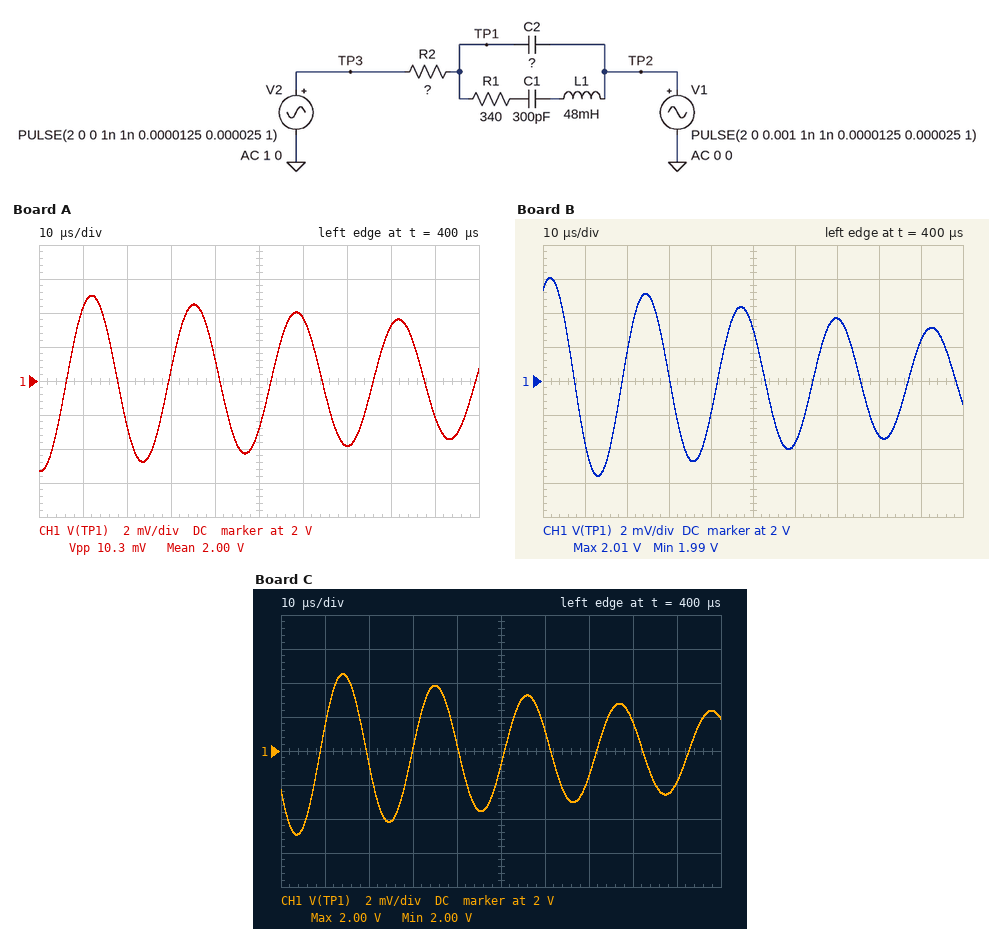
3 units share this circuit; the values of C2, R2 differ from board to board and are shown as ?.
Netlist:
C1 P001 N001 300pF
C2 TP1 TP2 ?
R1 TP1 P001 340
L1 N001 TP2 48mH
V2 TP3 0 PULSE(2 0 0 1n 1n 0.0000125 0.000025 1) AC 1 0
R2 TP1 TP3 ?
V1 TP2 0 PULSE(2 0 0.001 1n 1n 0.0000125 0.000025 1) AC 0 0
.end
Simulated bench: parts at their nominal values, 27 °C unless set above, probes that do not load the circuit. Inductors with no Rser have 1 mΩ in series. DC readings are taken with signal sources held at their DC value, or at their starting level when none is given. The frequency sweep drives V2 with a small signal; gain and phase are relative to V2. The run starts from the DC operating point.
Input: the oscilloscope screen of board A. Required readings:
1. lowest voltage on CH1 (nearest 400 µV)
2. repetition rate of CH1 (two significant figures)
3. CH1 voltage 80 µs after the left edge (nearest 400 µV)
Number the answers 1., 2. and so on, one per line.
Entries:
1. 1.9948 V
2. 43 kHz
3. 2.0032 V
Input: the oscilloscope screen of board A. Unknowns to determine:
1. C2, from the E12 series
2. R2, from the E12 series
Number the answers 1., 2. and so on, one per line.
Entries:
1. 5.6 nF
2. 3.9 kΩ
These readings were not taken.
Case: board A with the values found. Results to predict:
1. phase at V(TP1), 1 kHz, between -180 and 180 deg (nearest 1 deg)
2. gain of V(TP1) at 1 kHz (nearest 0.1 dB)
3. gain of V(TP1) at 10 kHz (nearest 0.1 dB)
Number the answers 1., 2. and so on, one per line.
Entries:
1. -8 deg
2. -0.1 dB
3. -4.9 dB
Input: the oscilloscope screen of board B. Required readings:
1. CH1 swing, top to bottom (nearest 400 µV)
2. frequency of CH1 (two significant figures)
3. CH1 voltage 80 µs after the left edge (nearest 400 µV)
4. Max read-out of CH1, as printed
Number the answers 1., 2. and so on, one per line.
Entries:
1. 11.6 mV
2. 44 kHz
3. 1.9968 V
4. 2.01 V
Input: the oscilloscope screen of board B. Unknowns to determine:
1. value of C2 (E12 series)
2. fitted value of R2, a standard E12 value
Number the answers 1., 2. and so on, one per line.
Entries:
1. 2.7 nF
2. 4.7 kΩ
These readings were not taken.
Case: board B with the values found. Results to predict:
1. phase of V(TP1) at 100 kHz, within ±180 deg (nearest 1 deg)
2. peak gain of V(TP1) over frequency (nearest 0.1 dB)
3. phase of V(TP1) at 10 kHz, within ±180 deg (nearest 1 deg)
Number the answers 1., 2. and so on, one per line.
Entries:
1. -83 deg
2. 0 dB
3. -42 deg
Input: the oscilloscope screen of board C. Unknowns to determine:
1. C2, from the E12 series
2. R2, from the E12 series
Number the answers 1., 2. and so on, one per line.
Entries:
1. 1 nF
2. 27 kΩ
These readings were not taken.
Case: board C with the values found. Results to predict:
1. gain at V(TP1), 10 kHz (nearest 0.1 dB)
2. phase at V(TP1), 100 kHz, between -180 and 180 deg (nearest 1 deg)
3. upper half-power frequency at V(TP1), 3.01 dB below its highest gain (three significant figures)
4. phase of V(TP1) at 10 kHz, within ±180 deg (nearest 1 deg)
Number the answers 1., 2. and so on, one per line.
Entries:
1. -7.8 dB
2. -86 deg
3. 4.52 kHz
4. -66 deg
